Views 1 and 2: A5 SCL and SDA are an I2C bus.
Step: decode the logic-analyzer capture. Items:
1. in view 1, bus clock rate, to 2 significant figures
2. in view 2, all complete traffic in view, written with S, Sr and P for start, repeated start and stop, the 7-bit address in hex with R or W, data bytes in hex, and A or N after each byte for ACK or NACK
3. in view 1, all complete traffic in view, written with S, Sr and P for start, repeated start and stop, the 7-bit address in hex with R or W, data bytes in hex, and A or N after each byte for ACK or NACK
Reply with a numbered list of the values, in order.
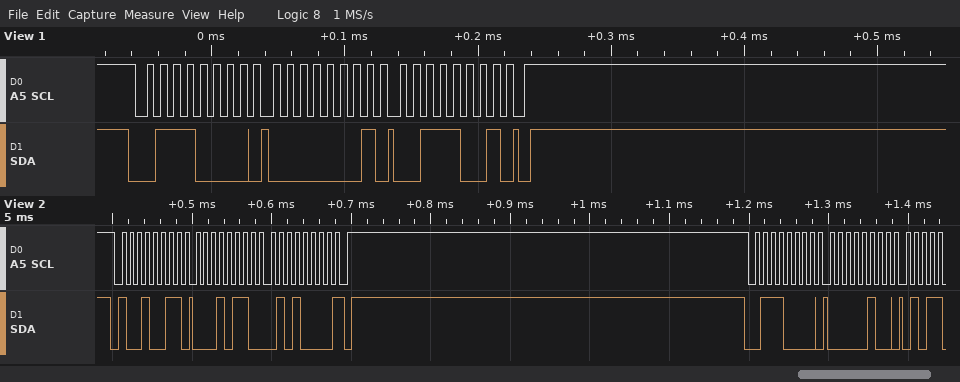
1. 100 kHz
2. S 49R A 16 A 50 N P S 38W A 04 A
3. S 38W A 01 A 39 A P
